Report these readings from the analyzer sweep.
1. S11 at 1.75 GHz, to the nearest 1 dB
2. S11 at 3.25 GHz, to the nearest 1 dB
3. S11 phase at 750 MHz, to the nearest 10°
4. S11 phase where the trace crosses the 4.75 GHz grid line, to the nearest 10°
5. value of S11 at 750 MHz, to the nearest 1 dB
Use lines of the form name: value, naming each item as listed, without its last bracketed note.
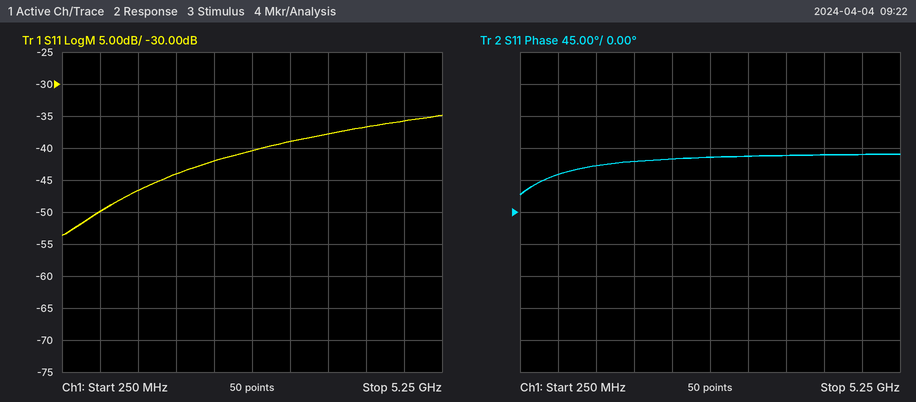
S11 at 1.75 GHz, to the nearest 1 dB: -44 dB
S11 at 3.25 GHz, to the nearest 1 dB: -39 dB
S11 phase at 750 MHz, to the nearest 10°: 50°
S11 phase where the trace crosses the 4.75 GHz grid line, to the nearest 10°: 80°
value of S11 at 750 MHz, to the nearest 1 dB: -50 dB
